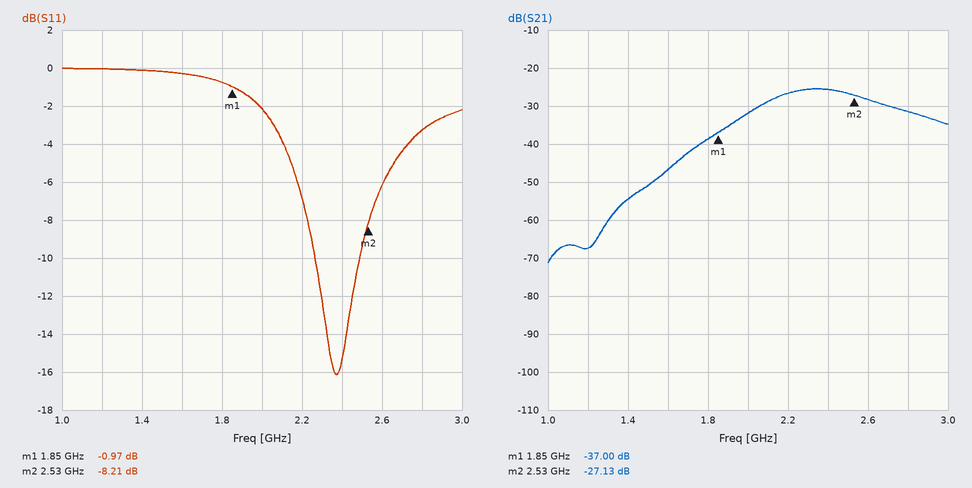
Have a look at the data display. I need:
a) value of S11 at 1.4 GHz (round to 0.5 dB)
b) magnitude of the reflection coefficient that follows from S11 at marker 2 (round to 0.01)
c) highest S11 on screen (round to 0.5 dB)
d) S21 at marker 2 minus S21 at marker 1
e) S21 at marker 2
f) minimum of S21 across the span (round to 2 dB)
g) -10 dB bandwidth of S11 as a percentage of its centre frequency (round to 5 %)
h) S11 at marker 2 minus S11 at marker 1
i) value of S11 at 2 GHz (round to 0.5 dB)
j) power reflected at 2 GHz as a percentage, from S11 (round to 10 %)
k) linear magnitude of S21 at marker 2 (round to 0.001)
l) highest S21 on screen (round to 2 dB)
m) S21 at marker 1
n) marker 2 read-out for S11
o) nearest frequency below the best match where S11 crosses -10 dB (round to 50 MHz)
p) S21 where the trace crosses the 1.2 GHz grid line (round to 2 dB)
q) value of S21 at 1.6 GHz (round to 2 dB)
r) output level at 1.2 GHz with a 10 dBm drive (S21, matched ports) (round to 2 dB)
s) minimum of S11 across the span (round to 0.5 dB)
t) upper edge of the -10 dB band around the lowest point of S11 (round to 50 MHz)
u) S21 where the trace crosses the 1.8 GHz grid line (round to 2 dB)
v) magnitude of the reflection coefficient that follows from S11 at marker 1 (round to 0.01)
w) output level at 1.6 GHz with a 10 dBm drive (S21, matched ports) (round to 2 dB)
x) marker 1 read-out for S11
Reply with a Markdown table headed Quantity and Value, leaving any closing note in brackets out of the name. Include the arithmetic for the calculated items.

| Quantity | Value |
|---|---|
| value of S11 at 1.4 GHz | 0.0 dB |
| magnitude of the reflection coefficient that follows from S11 at marker 2 | 10^(-8.21/20) ≈ 0.39 |
| highest S11 on screen | 0.0 dB |
| S21 at marker 2 minus S21 at marker 1 | -27.13 − (-37) = 9.87 dB |
| S21 at marker 2 | -27.13 dB |
| minimum of S21 across the span | -72 dB |
| -10 dB bandwidth of S11 as a percentage of its centre frequency | 250 MHz / 2.375 GHz ≈ 10 % |
| S11 at marker 2 minus S11 at marker 1 | -8.21 − (-0.97) = -7.24 dB |
| value of S11 at 2 GHz | -2.0 dB |
| power reflected at 2 GHz as a percentage, from S11 | 10^(-2/10) ≈ 63.1 %, so 60 % to the nearest 10 % |
| linear magnitude of S21 at marker 2 | 10^(-27.13/20) ≈ 0.044 |
| highest S21 on screen | -26 dB |
| S21 at marker 1 | -37.00 dB |
| marker 2 read-out for S11 | -8.21 dB |
| nearest frequency below the best match where S11 crosses -10 dB | 2.25 GHz |
| S21 where the trace crosses the 1.2 GHz grid line | -68 dB |
| value of S21 at 1.6 GHz | -46 dB |
| output level at 1.2 GHz with a 10 dBm drive (S21, matched ports) | 10 dBm + (-68 dB) = -58 dBm |
| minimum of S11 across the span | -16.0 dB |
| upper edge of the -10 dB band around the lowest point of S11 | 2.50 GHz |
| S21 where the trace crosses the 1.8 GHz grid line | -38 dB |
| magnitude of the reflection coefficient that follows from S11 at marker 1 | 10^(-0.97/20) ≈ 0.89 |
| output level at 1.6 GHz with a 10 dBm drive (S21, matched ports) | 10 dBm + (-46 dB) = -36 dBm |
| marker 1 read-out for S11 | -0.97 dB |
